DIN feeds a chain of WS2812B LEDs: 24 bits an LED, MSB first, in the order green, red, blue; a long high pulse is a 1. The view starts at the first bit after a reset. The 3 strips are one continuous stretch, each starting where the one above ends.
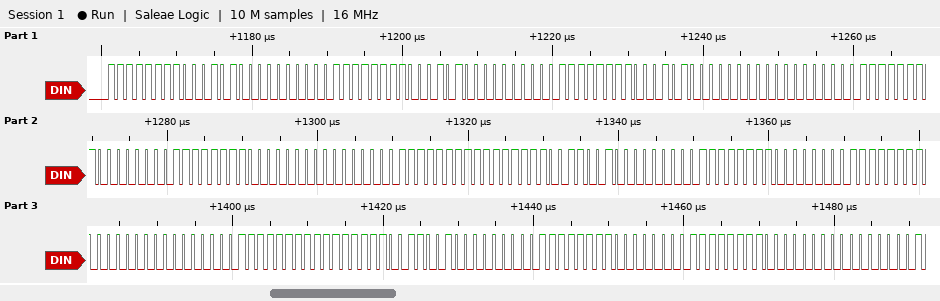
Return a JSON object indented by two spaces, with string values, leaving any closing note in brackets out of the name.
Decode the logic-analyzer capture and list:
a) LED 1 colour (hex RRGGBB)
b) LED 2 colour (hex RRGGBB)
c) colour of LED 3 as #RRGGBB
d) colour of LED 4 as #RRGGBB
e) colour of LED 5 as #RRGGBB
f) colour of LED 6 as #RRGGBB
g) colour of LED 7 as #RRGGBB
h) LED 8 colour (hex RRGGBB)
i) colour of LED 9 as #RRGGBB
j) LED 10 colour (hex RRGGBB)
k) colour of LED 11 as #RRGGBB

{
  "LED 1 colour": "#14FF00",
  "LED 2 colour": "#14FF00",
  "colour of LED 3 as #RRGGBB": "#14FF00",
  "colour of LED 4 as #RRGGBB": "#FF0000",
  "colour of LED 5 as #RRGGBB": "#00FF00",
  "colour of LED 6 as #RRGGBB": "#FFFF32",
  "colour of LED 7 as #RRGGBB": "#FF0000",
  "LED 8 colour": "#00FF00",
  "colour of LED 9 as #RRGGBB": "#FFFF32",
  "LED 10 colour": "#FF0000",
  "colour of LED 11 as #RRGGBB": "#00FF00"
}
